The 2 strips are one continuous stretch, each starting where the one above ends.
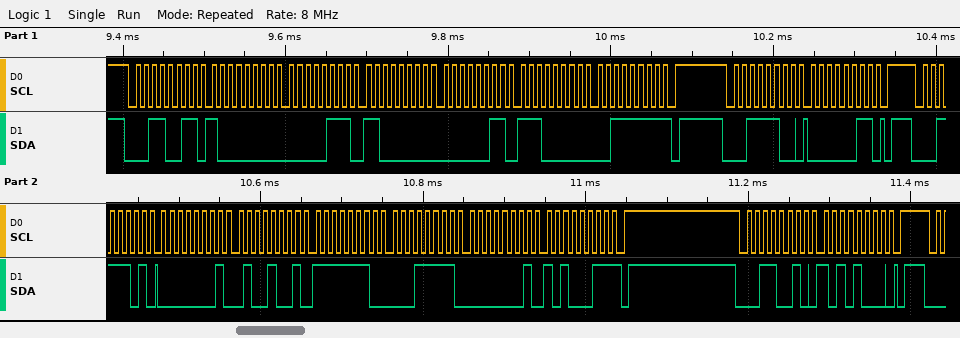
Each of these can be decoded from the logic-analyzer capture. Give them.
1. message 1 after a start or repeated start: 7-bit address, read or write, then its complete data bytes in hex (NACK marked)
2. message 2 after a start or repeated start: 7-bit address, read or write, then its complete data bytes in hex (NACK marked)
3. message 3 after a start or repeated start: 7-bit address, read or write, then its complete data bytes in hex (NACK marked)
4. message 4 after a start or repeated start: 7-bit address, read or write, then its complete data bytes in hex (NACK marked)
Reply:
0x19 read: 80 07 C0 03 E0 3F NACK
0x1E write: 03
0x1E read: 01 49 FE 1F 01 A3 NACK
0x19 write: A8
